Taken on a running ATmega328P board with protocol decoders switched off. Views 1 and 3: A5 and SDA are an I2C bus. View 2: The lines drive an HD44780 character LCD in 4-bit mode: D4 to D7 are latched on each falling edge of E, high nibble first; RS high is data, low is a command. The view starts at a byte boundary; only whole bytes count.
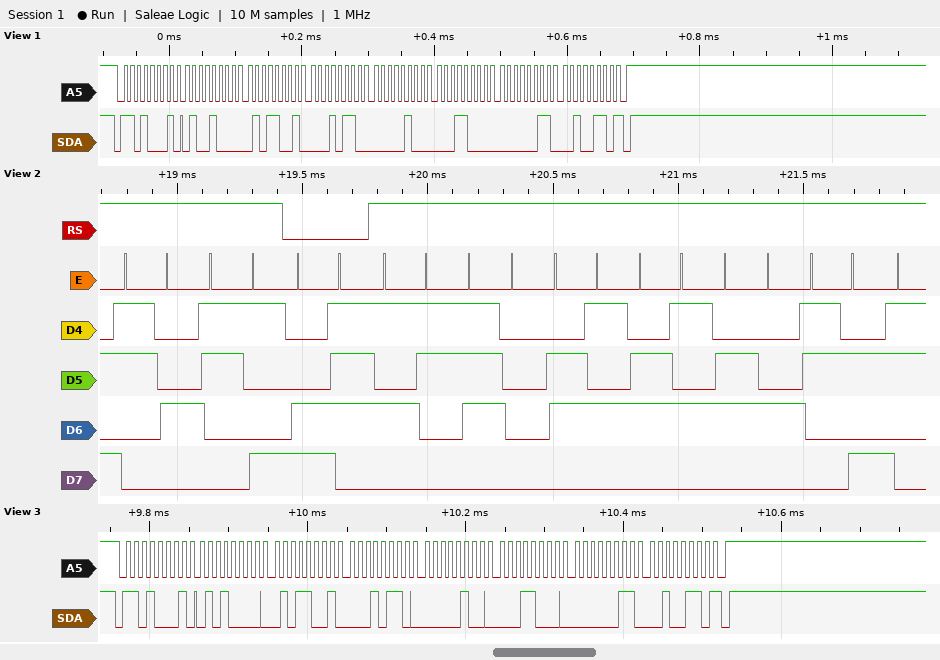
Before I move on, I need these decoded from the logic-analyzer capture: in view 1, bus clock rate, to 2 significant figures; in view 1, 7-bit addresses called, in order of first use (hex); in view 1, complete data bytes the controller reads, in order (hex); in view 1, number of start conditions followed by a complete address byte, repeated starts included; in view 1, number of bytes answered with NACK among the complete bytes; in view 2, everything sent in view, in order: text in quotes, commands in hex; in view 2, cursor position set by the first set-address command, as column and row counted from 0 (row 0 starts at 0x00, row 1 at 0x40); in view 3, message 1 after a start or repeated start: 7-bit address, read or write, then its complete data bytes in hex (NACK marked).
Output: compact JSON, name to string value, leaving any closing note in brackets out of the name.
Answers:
{"in view 1, bus clock rate, to 2 significant figures": "100 kHz", "in view 1, 7-bit addresses called, in order of first use": "0x68", "in view 1, complete data bytes the controller reads, in order": "48 59 16 04 18 03 26", "in view 1, number of start conditions followed by a complete address byte, repeated starts included": "1", "in view 1, number of bytes answered with NACK among the complete bytes": "1", "in view 2, everything sent in view, in order: text in quotes, commands in hex": "\"49\" 0xC7 \"Speed:\"", "in view 2, cursor position set by the first set-address command, as column and row counted from 0": "column 7, row 1", "in view 3, message 1 after a start or repeated start: 7-bit address, read or write, then its complete data bytes in hex": "0x68 read: 50 59 16 04 18 03 26 NACK"}
